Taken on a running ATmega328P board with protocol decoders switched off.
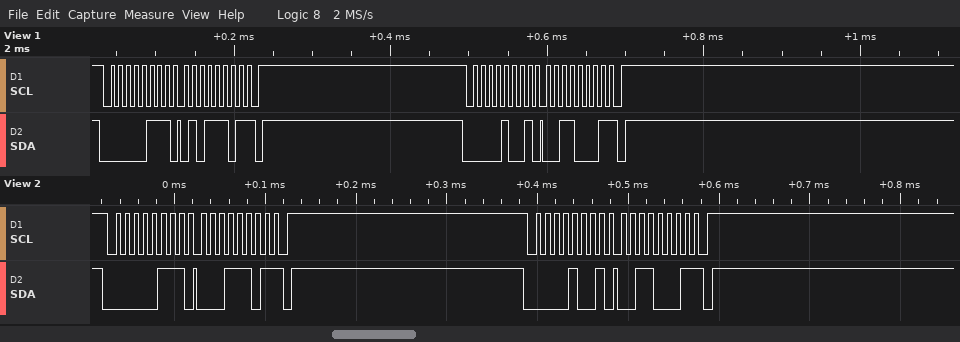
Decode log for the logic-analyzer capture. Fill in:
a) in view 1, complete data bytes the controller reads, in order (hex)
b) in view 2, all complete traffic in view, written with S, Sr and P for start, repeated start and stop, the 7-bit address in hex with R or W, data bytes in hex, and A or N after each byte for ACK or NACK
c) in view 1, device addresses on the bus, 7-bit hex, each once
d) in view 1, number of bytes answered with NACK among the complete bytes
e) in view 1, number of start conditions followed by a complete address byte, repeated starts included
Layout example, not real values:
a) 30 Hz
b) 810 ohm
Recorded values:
a) 5D 31
b) S 03R A 1D N P S 04R A 31 N P
c) 0x03 0x04
d) 2
e) 2
